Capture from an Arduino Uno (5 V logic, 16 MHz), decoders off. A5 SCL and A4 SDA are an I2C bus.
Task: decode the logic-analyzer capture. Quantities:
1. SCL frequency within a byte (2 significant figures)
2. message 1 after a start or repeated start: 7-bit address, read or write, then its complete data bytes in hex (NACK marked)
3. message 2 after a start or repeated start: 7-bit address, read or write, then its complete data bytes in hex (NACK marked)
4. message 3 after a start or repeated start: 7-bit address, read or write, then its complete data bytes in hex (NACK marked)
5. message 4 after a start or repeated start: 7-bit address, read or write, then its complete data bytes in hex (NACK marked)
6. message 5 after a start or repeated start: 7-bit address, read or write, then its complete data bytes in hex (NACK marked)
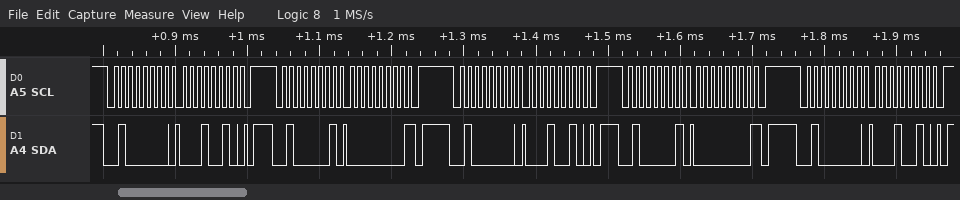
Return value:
100 kHz
0x20 write: 12
0x20 read: 00 NACK
0x20 write: 12
0x20 read: 00 NACK
0x20 write: 12
